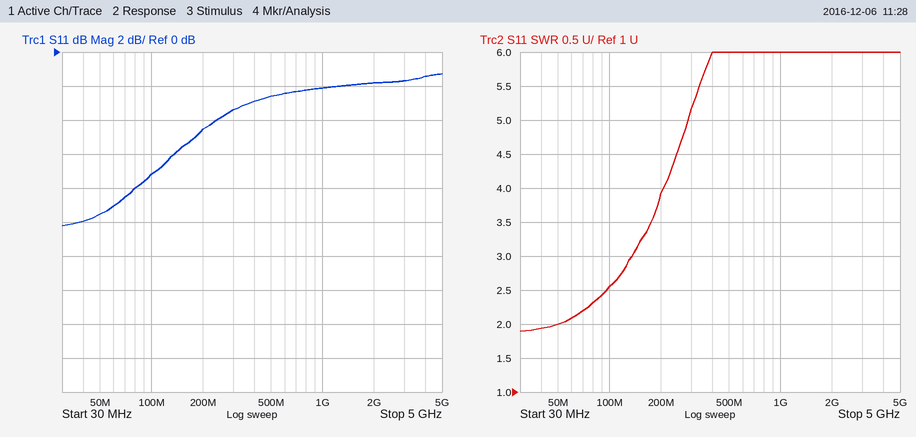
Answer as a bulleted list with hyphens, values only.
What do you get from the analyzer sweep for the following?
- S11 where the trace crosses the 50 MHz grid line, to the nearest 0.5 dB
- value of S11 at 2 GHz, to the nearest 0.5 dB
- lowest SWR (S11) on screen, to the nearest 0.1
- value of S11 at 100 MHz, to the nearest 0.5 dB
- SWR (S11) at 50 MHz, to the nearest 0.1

- -9.5 dB
- -2.0 dB
- 1.9
- -7.0 dB
- 2.0
